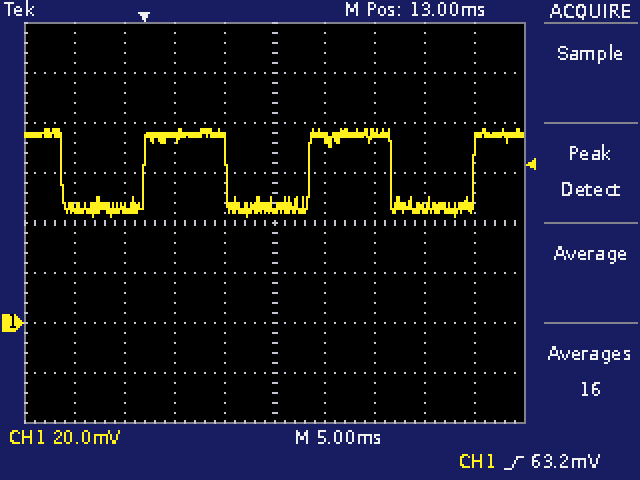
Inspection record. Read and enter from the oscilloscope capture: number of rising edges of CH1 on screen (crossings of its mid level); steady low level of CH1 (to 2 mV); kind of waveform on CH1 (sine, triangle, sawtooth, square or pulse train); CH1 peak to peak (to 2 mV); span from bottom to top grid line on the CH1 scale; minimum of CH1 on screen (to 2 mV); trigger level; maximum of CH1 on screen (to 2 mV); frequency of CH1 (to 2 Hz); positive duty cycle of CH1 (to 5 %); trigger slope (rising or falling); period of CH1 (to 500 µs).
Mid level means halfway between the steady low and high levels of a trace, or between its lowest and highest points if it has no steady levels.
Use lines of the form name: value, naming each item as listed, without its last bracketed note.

number of rising edges of CH1 on screen: 3
steady low level of CH1: 46 mV
kind of waveform on CH1: square
CH1 peak to peak: 36 mV
span from bottom to top grid line on the CH1 scale: 160 mV
minimum of CH1 on screen: 42 mV
trigger level: 63.2 mV
maximum of CH1 on screen: 78 mV
frequency of CH1: 60 Hz
positive duty cycle of CH1: 50 %
trigger slope: rising
period of CH1: 16.5 ms
